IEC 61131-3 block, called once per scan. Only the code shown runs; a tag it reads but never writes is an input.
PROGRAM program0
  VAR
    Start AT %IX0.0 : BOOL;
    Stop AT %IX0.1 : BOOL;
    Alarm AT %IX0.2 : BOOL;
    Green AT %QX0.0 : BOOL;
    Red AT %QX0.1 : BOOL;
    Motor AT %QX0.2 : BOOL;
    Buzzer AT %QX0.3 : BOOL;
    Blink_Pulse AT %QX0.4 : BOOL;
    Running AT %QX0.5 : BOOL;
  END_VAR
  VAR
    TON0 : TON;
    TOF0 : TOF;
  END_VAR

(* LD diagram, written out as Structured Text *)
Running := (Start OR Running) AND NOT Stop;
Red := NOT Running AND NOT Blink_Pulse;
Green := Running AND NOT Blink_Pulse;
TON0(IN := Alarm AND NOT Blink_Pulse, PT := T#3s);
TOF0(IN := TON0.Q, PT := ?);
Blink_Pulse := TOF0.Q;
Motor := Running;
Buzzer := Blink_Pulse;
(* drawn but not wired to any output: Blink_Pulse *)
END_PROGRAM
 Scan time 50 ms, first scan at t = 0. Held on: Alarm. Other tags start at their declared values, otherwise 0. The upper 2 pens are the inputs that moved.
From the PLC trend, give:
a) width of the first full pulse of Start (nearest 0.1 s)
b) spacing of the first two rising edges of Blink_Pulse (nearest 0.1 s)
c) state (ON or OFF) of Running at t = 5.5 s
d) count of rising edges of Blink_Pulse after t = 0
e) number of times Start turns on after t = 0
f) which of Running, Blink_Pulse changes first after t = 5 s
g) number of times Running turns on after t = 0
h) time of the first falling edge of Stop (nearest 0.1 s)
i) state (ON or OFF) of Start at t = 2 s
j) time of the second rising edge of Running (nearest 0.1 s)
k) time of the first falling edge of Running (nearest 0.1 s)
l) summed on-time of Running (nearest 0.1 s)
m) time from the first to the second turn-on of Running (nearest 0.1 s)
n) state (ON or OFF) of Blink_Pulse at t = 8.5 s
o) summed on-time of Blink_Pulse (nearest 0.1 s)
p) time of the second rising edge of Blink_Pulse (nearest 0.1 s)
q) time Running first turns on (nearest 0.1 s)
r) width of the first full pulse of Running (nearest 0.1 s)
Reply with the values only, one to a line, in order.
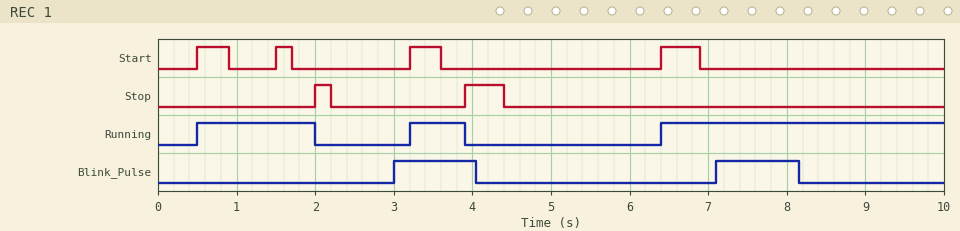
0.4 s
4.1 s
OFF
2
4
Running
3
2.2 s
OFF
3.2 s
2.0 s
5.8 s
2.7 s
OFF
2.1 s
7.1 s
0.5 s
1.5 s
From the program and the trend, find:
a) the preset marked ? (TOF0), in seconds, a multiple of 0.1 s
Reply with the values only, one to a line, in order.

1.0 s
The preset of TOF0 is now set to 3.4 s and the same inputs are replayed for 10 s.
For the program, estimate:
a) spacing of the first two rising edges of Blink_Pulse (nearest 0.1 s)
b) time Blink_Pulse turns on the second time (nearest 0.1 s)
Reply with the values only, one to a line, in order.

6.5 s
9.5 s
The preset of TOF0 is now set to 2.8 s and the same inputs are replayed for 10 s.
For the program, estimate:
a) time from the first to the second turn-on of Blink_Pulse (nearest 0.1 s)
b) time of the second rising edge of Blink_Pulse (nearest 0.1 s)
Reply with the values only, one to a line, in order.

5.9 s
8.9 s
